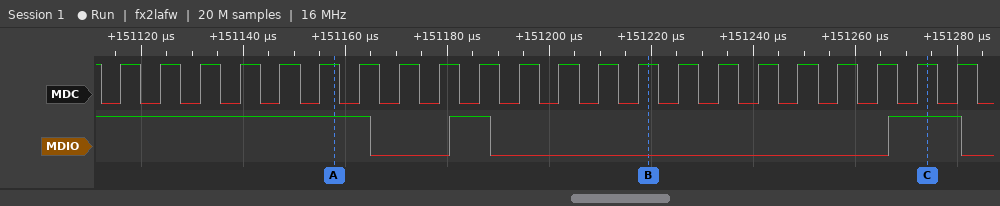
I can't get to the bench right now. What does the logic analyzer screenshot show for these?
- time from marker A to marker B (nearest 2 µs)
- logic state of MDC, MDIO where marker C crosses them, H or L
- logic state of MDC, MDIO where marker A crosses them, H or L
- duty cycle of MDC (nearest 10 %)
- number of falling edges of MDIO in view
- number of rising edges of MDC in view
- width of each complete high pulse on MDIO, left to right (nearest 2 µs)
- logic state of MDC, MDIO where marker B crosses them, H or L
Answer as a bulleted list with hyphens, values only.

- 62 µs
- MDC=H, MDIO=H
- MDC=H, MDIO=H
- 50 %
- 3
- 22
- 8 µs, 14 µs
- MDC=H, MDIO=L
